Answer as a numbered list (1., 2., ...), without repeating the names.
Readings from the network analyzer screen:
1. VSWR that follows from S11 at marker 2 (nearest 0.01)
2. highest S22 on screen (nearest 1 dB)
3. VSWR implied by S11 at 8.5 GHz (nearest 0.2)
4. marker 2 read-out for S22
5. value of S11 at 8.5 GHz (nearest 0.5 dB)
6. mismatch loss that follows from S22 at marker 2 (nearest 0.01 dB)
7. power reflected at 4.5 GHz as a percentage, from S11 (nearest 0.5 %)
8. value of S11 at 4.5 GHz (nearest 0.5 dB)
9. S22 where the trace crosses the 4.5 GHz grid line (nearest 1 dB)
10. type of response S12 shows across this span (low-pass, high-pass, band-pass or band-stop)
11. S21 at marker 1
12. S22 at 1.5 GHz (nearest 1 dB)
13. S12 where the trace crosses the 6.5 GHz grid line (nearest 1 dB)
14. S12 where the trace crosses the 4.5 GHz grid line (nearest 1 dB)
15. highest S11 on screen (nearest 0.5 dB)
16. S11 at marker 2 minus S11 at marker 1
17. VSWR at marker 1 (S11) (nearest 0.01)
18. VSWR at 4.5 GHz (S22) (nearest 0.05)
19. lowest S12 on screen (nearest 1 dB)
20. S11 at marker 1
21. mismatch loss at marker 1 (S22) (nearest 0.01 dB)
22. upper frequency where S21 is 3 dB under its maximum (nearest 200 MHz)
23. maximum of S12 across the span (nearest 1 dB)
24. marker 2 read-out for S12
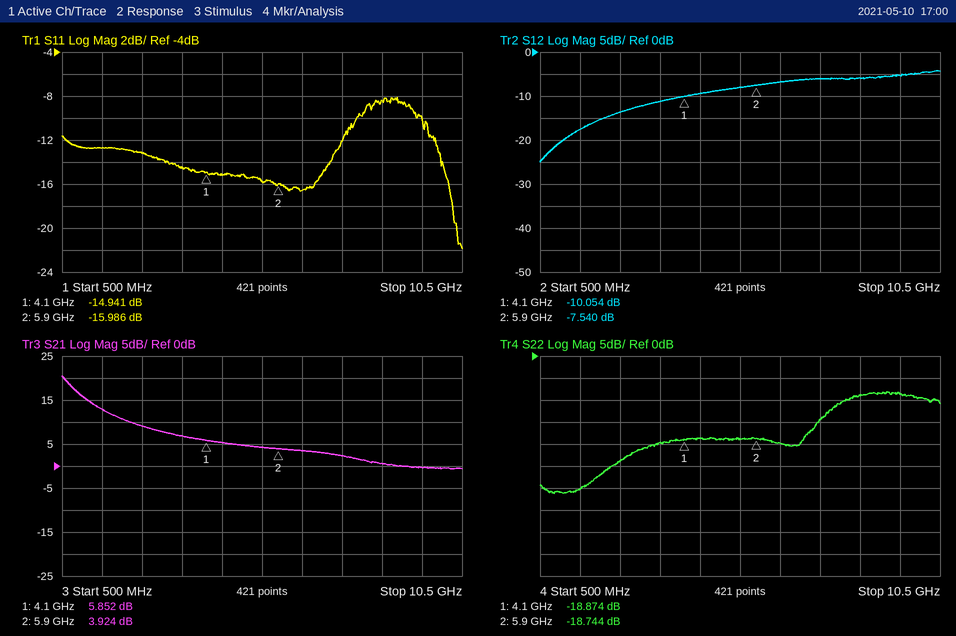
1. 1.38
2. -8 dB
3. 2.2
4. -18.744 dB
5. -8.5 dB
6. 0.06 dB
7. 3.0 %
8. -15.0 dB
9. -19 dB
10. high-pass
11. 5.852 dB
12. -30 dB
13. -7 dB
14. -9 dB
15. -8.0 dB
16. -1.045 dB
17. 1.44
18. 1.25
19. -25 dB
20. -14.941 dB
21. 0.06 dB
22. 800 MHz
23. -4 dB
24. -7.540 dB
